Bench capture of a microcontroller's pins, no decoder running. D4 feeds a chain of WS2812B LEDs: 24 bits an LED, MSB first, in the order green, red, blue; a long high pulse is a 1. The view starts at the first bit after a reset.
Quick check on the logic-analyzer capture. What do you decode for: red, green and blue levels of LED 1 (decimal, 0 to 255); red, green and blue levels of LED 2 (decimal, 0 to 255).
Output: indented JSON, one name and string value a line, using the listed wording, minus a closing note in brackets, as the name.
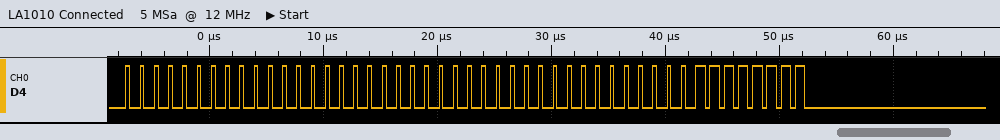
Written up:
{
  "red, green and blue levels of LED 1": "0, 0, 0",
  "red, green and blue levels of LED 2": "0, 0, 255"
}
